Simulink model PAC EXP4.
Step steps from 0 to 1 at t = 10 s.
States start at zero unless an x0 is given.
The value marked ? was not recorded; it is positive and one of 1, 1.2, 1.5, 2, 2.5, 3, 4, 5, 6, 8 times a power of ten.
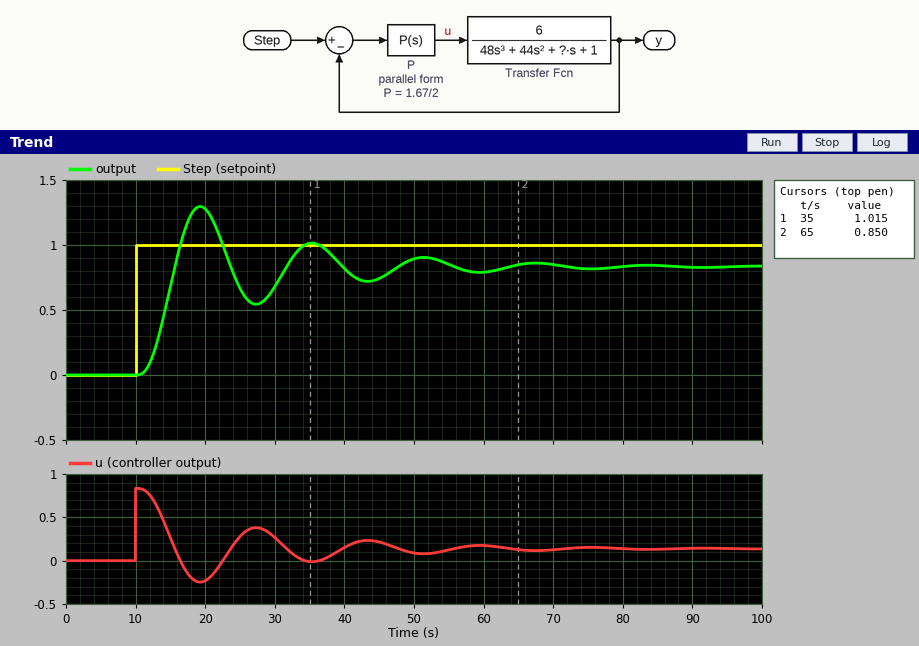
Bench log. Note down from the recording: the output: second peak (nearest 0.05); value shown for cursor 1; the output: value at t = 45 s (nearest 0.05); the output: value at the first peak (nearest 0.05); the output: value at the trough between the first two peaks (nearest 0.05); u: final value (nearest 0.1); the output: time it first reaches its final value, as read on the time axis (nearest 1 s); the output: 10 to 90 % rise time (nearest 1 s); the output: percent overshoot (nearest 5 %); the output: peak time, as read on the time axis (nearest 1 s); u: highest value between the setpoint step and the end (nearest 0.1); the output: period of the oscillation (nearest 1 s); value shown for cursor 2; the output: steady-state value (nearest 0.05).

1.00
1.015
0.75
1.30
0.55
0.1
16 s
3 s
55 %
19 s
0.8
16 s
0.850
0.85
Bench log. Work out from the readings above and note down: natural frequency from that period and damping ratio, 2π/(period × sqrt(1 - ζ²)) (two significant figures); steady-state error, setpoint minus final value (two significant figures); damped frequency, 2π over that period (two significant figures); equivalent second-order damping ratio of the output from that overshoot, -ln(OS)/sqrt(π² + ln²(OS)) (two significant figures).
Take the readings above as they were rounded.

0.40 rad/s
0.15
0.39 rad/s
0.19
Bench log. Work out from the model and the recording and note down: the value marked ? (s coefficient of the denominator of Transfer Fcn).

12
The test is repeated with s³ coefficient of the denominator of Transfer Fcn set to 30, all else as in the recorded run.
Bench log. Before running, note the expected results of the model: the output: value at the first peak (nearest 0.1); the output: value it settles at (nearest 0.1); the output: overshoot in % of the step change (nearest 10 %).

1.2
0.8
40 %
